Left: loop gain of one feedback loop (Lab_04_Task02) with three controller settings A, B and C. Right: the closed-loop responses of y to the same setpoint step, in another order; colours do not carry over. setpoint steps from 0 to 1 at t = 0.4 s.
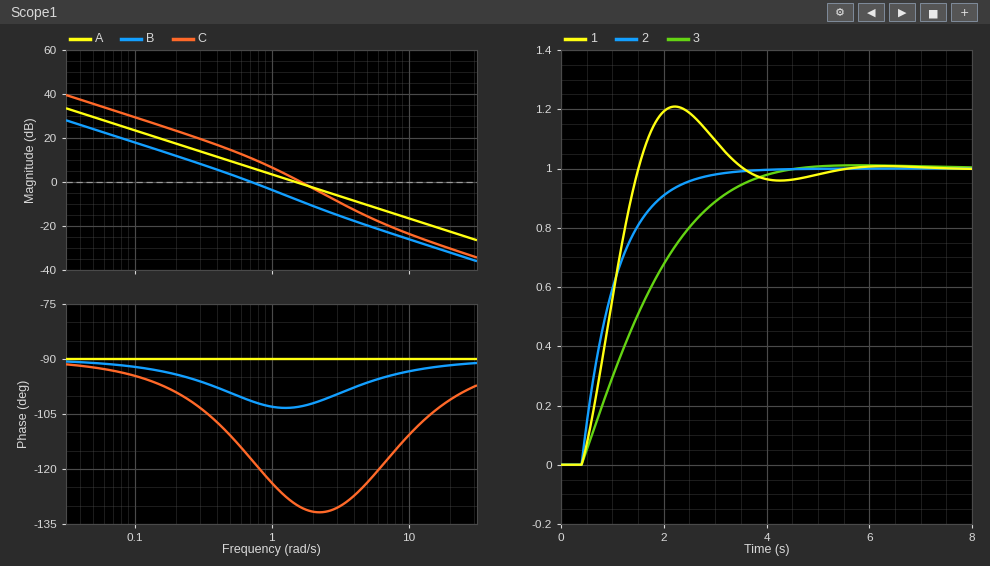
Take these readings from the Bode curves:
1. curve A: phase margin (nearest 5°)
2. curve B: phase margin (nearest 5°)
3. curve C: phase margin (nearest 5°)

90°
80°
50°
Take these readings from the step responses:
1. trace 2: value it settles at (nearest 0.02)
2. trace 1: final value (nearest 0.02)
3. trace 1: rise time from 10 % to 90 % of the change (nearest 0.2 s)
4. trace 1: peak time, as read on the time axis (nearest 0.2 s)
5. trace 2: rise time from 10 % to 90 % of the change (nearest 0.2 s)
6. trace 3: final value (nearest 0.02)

1.00
1.00
0.8 s
2.2 s
1.4 s
1.00
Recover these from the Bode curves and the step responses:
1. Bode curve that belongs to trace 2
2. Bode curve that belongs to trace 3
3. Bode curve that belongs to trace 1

A
B
C
